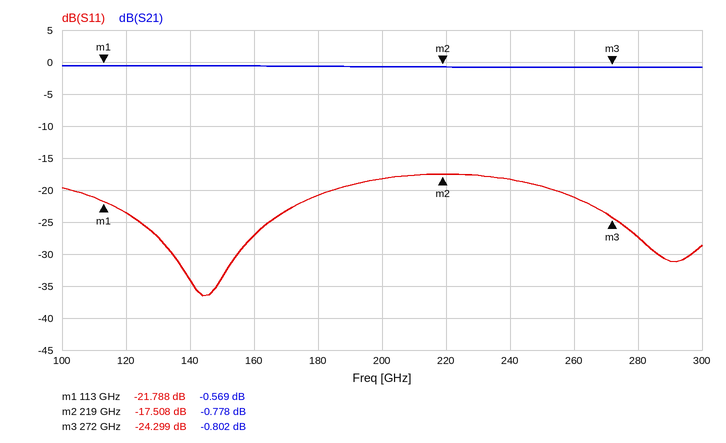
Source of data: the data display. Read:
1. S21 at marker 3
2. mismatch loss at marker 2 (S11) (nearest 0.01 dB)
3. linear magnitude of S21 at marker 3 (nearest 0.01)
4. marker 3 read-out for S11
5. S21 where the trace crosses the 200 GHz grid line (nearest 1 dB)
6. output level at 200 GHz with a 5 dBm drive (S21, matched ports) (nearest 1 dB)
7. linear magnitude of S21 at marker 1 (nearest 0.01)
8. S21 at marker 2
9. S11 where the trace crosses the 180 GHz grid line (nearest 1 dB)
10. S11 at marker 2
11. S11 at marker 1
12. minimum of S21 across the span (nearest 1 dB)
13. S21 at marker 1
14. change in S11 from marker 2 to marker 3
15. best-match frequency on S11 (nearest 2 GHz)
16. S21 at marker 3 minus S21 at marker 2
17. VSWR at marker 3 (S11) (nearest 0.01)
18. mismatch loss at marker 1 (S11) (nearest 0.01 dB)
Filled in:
-0.802 dB
0.08 dB
0.91
-24.299 dB
-1 dB
4 dBm
0.94
-0.778 dB
-21 dB
-17.508 dB
-21.788 dB
-1 dB
-0.569 dB
-6.791 dB
144 GHz
-0.024 dB
1.13
0.03 dB
